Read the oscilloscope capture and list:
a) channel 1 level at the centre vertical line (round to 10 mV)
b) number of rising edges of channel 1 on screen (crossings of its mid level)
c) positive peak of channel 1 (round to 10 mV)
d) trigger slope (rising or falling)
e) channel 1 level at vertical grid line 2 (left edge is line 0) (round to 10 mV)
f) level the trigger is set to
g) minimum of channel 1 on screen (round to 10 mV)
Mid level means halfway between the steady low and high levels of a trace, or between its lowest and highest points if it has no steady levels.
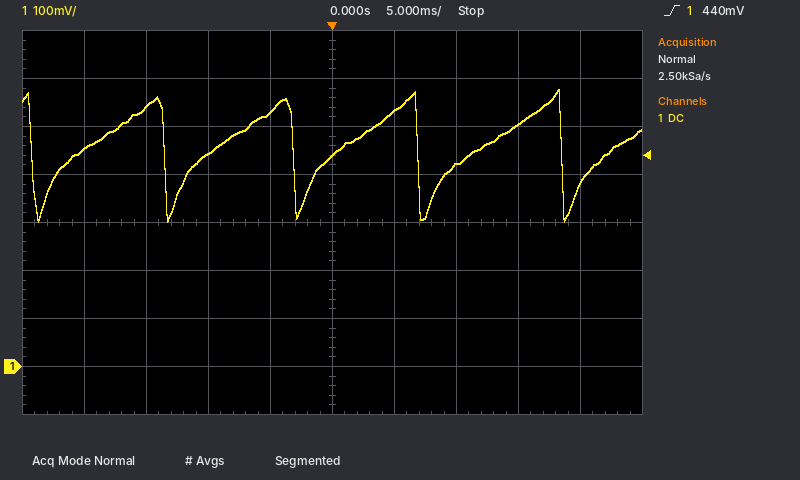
440 mV
5
580 mV
rising
540 mV
440 mV
300 mV
